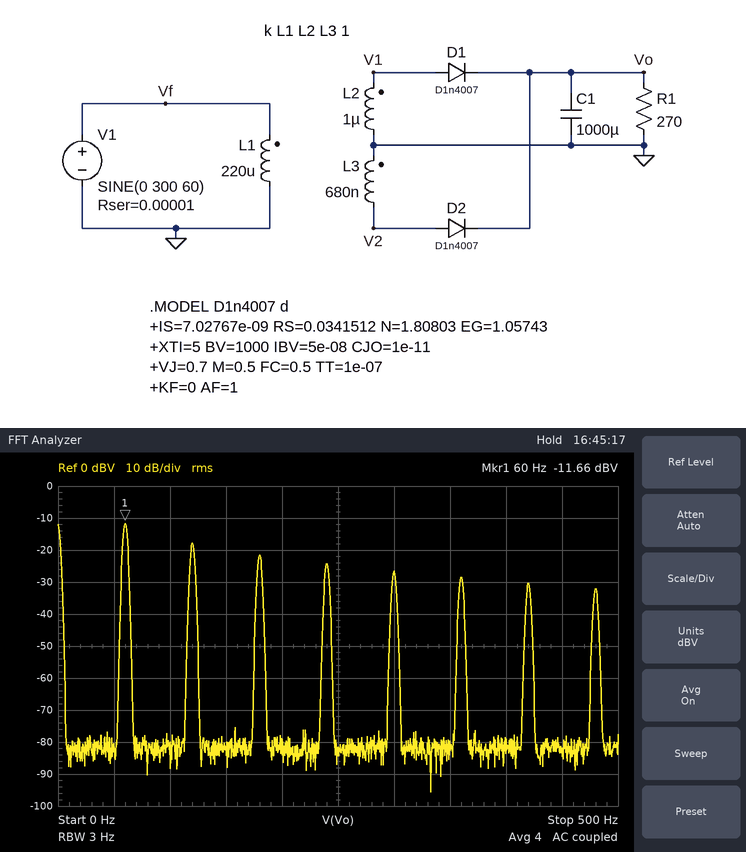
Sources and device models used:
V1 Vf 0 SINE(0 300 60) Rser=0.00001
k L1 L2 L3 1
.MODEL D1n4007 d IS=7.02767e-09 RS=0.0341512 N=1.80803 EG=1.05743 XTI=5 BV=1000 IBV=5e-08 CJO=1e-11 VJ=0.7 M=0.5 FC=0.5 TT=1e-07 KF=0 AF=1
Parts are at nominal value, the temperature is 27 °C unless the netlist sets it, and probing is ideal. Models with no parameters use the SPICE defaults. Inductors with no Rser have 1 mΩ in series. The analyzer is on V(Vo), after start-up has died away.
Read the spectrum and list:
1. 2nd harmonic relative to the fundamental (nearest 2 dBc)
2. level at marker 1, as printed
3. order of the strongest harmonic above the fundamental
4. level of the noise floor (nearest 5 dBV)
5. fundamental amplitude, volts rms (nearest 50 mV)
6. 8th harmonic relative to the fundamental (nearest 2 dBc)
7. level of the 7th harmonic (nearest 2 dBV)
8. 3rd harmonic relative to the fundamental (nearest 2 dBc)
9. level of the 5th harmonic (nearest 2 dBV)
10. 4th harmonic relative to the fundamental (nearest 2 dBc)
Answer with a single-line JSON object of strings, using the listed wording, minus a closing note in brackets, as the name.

{"2nd harmonic relative to the fundamental": "-6 dBc", "level at marker 1, as printed": "-11.66 dBV", "order of the strongest harmonic above the fundamental": "2", "level of the noise floor": "-80 dBV", "fundamental amplitude, volts rms": "250 mV", "8th harmonic relative to the fundamental": "-20 dBc", "level of the 7th harmonic": "-30 dBV", "3rd harmonic relative to the fundamental": "-10 dBc", "level of the 5th harmonic": "-26 dBV", "4th harmonic relative to the fundamental": "-12 dBc"}
